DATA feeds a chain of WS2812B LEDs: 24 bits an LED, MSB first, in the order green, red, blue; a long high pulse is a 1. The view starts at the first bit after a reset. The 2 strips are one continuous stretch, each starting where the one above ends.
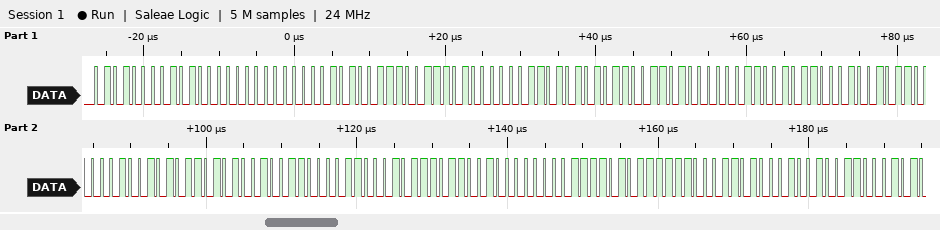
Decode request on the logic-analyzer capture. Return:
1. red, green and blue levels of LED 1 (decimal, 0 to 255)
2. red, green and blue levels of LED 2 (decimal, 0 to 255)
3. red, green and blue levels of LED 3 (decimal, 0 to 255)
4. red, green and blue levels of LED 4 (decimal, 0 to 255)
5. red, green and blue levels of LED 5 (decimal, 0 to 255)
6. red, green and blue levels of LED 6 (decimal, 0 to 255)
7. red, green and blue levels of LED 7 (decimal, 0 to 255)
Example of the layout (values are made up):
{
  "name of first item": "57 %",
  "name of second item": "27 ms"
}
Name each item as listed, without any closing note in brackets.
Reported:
{
  "red, green and blue levels of LED 1": "160, 80, 0",
  "red, green and blue levels of LED 2": "157, 83, 3",
  "red, green and blue levels of LED 3": "154, 85, 6",
  "red, green and blue levels of LED 4": "150, 88, 9",
  "red, green and blue levels of LED 5": "147, 90, 12",
  "red, green and blue levels of LED 6": "144, 93, 15",
  "red, green and blue levels of LED 7": "141, 95, 18"
}
